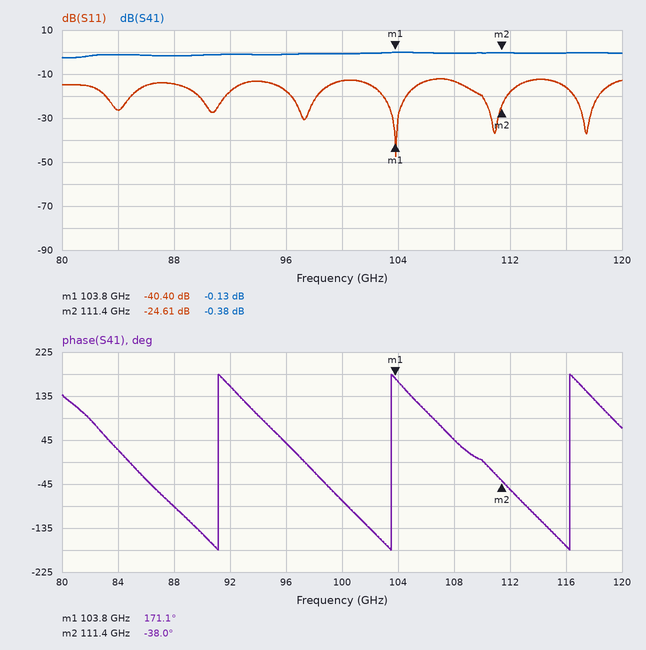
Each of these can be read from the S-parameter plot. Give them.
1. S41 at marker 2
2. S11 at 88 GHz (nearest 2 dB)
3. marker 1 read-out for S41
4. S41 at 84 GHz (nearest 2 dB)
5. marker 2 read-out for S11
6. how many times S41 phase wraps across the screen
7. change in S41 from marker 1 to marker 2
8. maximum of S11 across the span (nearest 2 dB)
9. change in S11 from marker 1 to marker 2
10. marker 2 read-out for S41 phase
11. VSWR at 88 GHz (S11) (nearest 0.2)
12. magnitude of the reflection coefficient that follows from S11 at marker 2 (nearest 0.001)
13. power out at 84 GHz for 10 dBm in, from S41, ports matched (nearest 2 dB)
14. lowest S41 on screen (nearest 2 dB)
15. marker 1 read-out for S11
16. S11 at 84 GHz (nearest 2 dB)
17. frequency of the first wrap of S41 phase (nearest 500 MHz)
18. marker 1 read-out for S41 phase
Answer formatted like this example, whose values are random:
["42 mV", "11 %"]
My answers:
["-0.38 dB", "-14 dB", "-0.13 dB", "-2 dB", "-24.61 dB", "3", "-0.25 dB", "-12 dB", "15.79 dB", "-38.0°", "1.4", "0.059", "8 dBm", "-2 dB", "-40.40 dB", "-26 dB", "91.0 GHz", "171.1°"]
